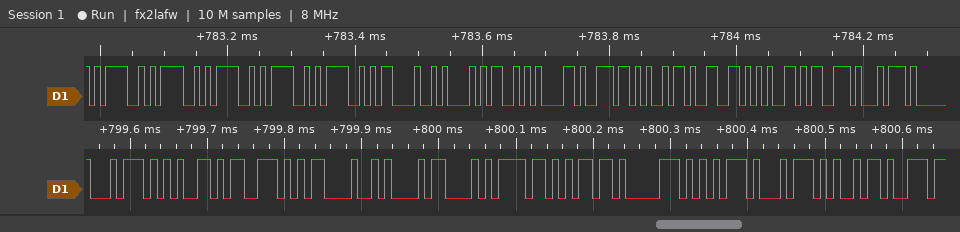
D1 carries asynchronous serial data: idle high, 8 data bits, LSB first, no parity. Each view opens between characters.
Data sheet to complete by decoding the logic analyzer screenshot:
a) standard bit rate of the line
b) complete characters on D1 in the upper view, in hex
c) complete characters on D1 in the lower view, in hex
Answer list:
115200 baud
3D, 3D, 3D, 3D, 3D, 0D, 0A, 4D, 61, 6E, 69, 66, 65, 73, 74
74, 65, 73, 0D, 0A, 43, 6F, 6D, 70, 75, 74, 69
